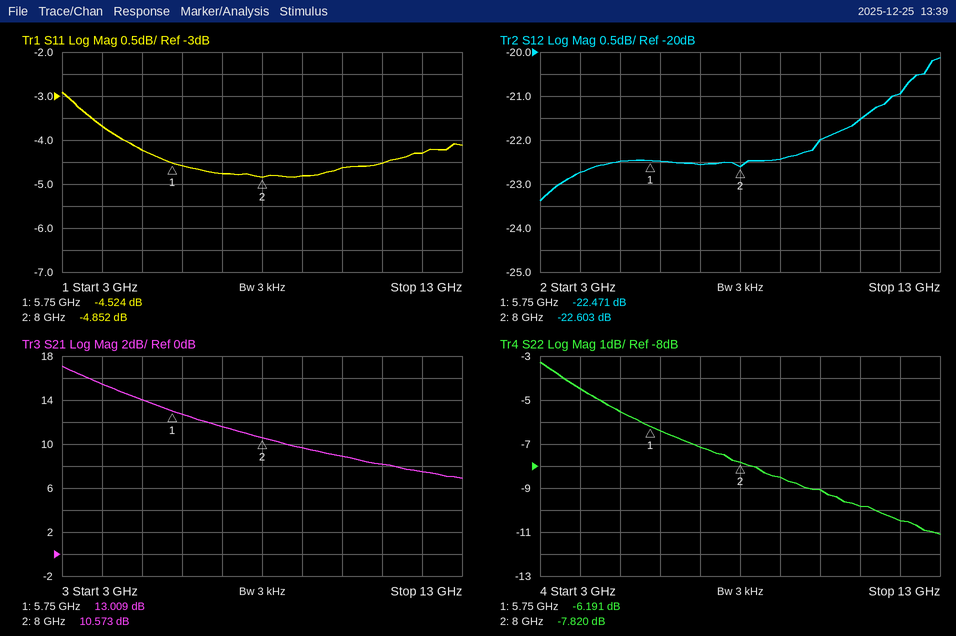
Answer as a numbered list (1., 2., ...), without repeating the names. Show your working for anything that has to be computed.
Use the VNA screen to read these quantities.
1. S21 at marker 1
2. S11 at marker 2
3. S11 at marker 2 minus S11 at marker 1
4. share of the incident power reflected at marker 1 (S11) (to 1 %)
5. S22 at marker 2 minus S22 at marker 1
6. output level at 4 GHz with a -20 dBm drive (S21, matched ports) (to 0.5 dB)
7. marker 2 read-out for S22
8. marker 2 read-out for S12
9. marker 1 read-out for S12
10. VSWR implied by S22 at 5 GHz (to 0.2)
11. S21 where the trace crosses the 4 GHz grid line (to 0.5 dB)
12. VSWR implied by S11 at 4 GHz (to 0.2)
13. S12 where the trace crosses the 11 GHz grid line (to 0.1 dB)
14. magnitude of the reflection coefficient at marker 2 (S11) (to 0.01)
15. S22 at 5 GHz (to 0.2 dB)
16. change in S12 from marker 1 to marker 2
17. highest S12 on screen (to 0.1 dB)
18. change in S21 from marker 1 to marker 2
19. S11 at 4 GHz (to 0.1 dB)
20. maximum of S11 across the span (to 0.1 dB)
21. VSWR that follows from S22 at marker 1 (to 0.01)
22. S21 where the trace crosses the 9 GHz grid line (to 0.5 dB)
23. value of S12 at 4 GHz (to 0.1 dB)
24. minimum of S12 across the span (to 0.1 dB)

1. 13.009 dB
2. -4.852 dB
3. -4.852 − (-4.524) = -0.328 dB
4. 10^(-4.524/10) ≈ 35 %
5. -7.82 − (-6.191) = -1.629 dB
6. -20 dBm + (15.5 dB) = -4.5 dBm
7. -7.820 dB
8. -22.603 dB
9. -22.471 dB
10. |Γ| = 10^(-5.6/20) = 0.5248; VSWR = (1 + 0.5248)/(1 − 0.5248) ≈ 3.2
11. 15.5 dB
12. |Γ| = 10^(-3.7/20) = 0.6531; VSWR = (1 + 0.6531)/(1 − 0.6531) ≈ 4.8
13. -21.5 dB
14. 10^(-4.852/20) ≈ 0.57
15. -5.6 dB
16. -22.603 − (-22.471) = -0.132 dB
17. -20.1 dB
18. 10.573 − (13.009) = -2.436 dB
19. -3.7 dB
20. -2.9 dB
21. (1 + 0.4903)/(1 − 0.4903) ≈ 2.92
22. 9.5 dB
23. -22.7 dB
24. -23.4 dB
